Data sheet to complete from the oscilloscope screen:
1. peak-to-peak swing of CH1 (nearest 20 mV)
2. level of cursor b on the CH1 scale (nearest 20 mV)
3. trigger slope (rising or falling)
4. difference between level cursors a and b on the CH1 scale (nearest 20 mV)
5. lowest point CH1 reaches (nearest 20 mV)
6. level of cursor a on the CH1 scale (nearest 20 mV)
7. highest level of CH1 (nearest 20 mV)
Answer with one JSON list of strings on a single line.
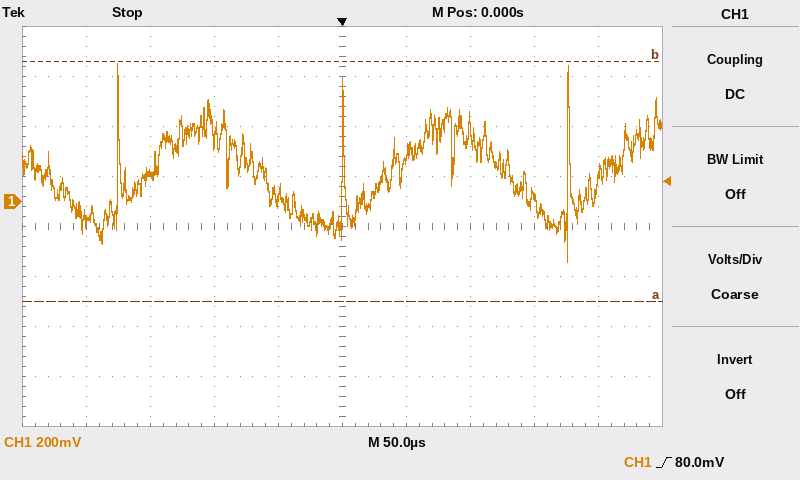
["800 mV", "560 mV", "rising", "960 mV", "-240 mV", "-400 mV", "560 mV"]
